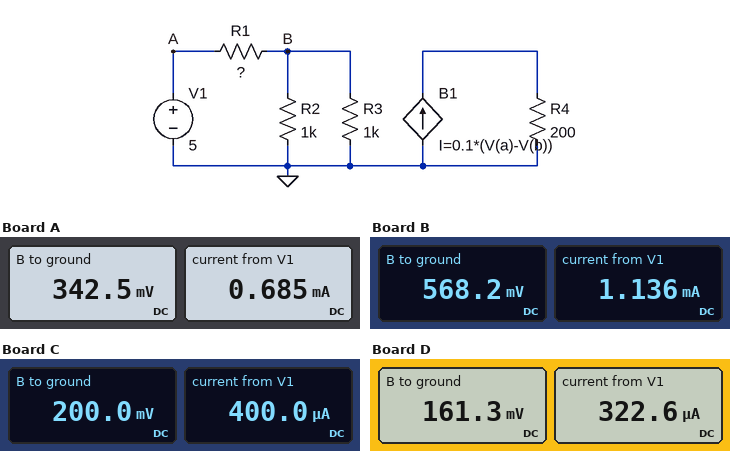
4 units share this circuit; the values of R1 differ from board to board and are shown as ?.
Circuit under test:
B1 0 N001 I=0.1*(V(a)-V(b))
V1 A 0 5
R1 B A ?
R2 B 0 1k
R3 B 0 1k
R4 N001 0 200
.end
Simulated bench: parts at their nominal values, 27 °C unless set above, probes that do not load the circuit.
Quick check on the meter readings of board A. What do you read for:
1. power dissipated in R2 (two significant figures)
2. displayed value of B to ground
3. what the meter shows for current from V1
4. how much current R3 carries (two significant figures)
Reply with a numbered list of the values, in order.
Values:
1. 120 µW
2. 342.5 mV
3. 0.685 mA
4. 340 µA
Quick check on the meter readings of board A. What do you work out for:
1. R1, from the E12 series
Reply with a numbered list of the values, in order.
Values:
1. 6.8 kΩ
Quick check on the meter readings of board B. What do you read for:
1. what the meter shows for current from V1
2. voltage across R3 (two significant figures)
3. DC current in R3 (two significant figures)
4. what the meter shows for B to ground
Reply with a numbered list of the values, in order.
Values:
1. 1.136 mA
2. 570 mV
3. 570 µA
4. 568.2 mV
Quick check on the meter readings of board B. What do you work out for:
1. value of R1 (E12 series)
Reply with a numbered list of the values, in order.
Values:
1. 3.9 kΩ
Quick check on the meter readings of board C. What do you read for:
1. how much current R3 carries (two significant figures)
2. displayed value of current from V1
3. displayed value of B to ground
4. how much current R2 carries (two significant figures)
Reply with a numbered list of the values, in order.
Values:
1. 200 µA
2. 400.0 µA
3. 200.0 mV
4. 200 µA
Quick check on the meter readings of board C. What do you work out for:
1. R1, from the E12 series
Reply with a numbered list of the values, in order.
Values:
1. 12 kΩ
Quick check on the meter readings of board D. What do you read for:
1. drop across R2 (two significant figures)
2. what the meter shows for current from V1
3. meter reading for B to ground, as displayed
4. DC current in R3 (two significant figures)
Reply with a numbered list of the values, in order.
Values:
1. 160 mV
2. 322.6 µA
3. 161.3 mV
4. 160 µA
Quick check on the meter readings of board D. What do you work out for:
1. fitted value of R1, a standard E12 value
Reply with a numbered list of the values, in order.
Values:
1. 15 kΩ
